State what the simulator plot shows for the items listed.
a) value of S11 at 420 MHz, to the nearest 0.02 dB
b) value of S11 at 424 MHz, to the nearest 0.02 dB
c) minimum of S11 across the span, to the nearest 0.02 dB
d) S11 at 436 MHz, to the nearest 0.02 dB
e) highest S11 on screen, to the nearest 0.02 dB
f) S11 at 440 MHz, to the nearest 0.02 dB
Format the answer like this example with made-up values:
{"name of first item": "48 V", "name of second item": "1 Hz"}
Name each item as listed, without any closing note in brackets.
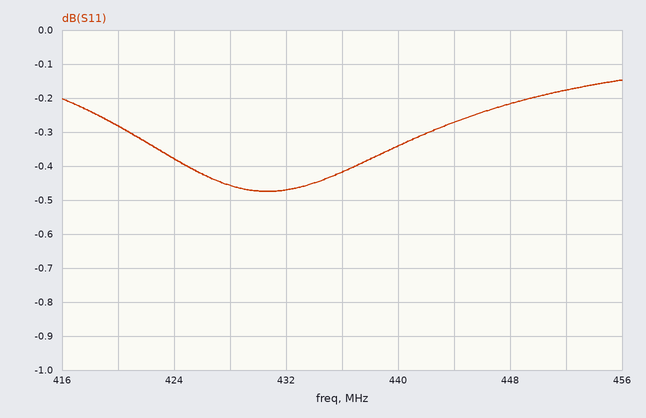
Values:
{"value of S11 at 420 MHz, to the nearest 0.02 dB": "-0.28 dB", "value of S11 at 424 MHz, to the nearest 0.02 dB": "-0.38 dB", "minimum of S11 across the span, to the nearest 0.02 dB": "-0.48 dB", "S11 at 436 MHz, to the nearest 0.02 dB": "-0.42 dB", "highest S11 on screen, to the nearest 0.02 dB": "-0.14 dB", "S11 at 440 MHz, to the nearest 0.02 dB": "-0.34 dB"}
